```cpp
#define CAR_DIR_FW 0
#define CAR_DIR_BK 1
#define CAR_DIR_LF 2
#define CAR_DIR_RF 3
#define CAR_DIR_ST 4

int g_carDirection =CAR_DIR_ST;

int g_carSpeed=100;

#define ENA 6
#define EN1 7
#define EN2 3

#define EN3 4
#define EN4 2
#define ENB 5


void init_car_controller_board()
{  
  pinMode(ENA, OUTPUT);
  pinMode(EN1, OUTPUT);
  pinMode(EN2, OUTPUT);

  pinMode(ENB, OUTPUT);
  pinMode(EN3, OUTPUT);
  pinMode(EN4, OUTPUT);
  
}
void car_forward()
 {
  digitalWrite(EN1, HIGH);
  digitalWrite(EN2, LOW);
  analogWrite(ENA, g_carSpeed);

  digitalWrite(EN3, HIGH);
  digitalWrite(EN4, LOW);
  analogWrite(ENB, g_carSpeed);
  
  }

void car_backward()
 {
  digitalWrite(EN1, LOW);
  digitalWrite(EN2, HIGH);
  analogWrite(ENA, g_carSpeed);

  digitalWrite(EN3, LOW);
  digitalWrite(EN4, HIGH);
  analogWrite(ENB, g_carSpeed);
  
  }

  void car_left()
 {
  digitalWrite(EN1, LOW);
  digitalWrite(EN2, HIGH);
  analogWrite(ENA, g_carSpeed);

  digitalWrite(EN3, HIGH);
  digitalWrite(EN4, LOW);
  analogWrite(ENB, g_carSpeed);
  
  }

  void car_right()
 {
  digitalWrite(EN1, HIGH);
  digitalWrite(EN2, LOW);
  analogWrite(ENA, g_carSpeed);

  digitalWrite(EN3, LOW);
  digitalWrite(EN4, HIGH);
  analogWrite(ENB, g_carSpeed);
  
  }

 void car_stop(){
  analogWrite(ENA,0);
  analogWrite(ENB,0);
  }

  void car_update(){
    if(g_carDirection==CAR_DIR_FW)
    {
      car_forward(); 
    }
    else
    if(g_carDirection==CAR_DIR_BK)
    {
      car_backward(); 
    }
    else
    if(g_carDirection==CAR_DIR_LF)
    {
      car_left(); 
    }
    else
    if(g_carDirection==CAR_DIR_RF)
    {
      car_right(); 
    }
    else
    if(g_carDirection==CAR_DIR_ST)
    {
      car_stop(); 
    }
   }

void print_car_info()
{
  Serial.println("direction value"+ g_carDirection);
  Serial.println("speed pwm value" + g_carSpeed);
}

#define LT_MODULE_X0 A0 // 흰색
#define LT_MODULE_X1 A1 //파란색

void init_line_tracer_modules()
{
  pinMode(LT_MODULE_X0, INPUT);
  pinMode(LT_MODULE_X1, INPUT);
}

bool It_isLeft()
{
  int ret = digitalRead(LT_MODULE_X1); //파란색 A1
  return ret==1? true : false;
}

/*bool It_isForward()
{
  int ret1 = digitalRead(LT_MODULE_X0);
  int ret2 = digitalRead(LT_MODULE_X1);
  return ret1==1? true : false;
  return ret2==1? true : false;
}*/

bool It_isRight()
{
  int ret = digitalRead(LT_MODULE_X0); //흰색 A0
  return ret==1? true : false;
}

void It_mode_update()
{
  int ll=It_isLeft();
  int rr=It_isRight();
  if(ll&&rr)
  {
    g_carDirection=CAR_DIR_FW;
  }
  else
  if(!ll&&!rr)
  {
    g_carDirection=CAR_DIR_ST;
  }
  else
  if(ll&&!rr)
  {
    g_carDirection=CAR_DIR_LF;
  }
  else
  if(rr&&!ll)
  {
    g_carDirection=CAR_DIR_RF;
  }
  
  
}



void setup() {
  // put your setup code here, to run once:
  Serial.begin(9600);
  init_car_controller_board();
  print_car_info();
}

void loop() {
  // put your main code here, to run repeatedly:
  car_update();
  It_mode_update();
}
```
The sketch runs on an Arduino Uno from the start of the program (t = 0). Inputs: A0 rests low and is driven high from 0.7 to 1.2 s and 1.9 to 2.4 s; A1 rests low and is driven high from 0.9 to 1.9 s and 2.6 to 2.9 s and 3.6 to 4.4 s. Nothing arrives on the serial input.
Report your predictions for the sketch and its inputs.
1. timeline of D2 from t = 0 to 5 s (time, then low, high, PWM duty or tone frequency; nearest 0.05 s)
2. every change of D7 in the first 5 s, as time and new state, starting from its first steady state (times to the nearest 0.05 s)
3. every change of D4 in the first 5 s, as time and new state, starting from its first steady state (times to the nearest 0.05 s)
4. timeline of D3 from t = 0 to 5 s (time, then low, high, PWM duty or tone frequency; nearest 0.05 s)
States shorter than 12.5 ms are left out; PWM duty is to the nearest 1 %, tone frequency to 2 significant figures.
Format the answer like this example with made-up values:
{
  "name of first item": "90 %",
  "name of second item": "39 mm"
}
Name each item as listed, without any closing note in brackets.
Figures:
{
  "timeline of D2 from t = 0 to 5 s": "0 s low; 0.7 s high; 0.9 s low; 1.9 s high; 2.6 s low",
  "every change of D7 in the first 5 s, as time and new state, starting from its first steady state": "0 s low; 0.7 s high; 1.2 s low; 1.9 s high; 2.6 s low",
  "every change of D4 in the first 5 s, as time and new state, starting from its first steady state": "0 s low; 0.9 s high; 1.9 s low; 2.6 s high",
  "timeline of D3 from t = 0 to 5 s": "0 s low; 1.2 s high; 1.9 s low; 2.6 s high"
}
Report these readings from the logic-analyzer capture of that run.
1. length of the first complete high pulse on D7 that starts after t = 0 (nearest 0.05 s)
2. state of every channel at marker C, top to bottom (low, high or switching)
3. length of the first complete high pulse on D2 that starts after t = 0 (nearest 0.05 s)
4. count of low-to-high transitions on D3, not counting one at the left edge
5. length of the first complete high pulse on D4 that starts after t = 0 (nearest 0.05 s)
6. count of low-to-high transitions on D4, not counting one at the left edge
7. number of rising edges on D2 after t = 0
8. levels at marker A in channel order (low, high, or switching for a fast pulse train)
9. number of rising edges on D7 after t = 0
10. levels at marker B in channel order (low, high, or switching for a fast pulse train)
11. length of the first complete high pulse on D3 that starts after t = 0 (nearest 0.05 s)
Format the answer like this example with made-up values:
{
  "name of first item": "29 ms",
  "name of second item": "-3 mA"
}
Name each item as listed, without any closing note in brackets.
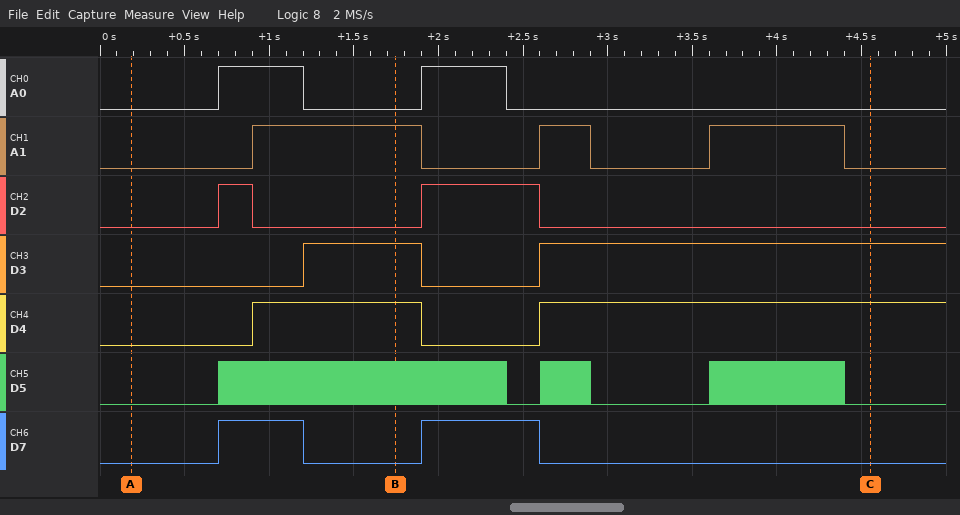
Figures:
{
  "length of the first complete high pulse on D7 that starts after t = 0": "0.50 s",
  "state of every channel at marker C, top to bottom": "A0 low, A1 low, D2 low, D3 high, D4 high, D5 low, D7 low",
  "length of the first complete high pulse on D2 that starts after t = 0": "0.20 s",
  "count of low-to-high transitions on D3, not counting one at the left edge": "2",
  "length of the first complete high pulse on D4 that starts after t = 0": "1.00 s",
  "count of low-to-high transitions on D4, not counting one at the left edge": "2",
  "number of rising edges on D2 after t = 0": "2",
  "levels at marker A in channel order": "A0 low, A1 low, D2 low, D3 low, D4 low, D5 low, D7 low",
  "number of rising edges on D7 after t = 0": "2",
  "levels at marker B in channel order": "A0 low, A1 high, D2 low, D3 high, D4 high, D5 switching, D7 low",
  "length of the first complete high pulse on D3 that starts after t = 0": "0.70 s"
}
